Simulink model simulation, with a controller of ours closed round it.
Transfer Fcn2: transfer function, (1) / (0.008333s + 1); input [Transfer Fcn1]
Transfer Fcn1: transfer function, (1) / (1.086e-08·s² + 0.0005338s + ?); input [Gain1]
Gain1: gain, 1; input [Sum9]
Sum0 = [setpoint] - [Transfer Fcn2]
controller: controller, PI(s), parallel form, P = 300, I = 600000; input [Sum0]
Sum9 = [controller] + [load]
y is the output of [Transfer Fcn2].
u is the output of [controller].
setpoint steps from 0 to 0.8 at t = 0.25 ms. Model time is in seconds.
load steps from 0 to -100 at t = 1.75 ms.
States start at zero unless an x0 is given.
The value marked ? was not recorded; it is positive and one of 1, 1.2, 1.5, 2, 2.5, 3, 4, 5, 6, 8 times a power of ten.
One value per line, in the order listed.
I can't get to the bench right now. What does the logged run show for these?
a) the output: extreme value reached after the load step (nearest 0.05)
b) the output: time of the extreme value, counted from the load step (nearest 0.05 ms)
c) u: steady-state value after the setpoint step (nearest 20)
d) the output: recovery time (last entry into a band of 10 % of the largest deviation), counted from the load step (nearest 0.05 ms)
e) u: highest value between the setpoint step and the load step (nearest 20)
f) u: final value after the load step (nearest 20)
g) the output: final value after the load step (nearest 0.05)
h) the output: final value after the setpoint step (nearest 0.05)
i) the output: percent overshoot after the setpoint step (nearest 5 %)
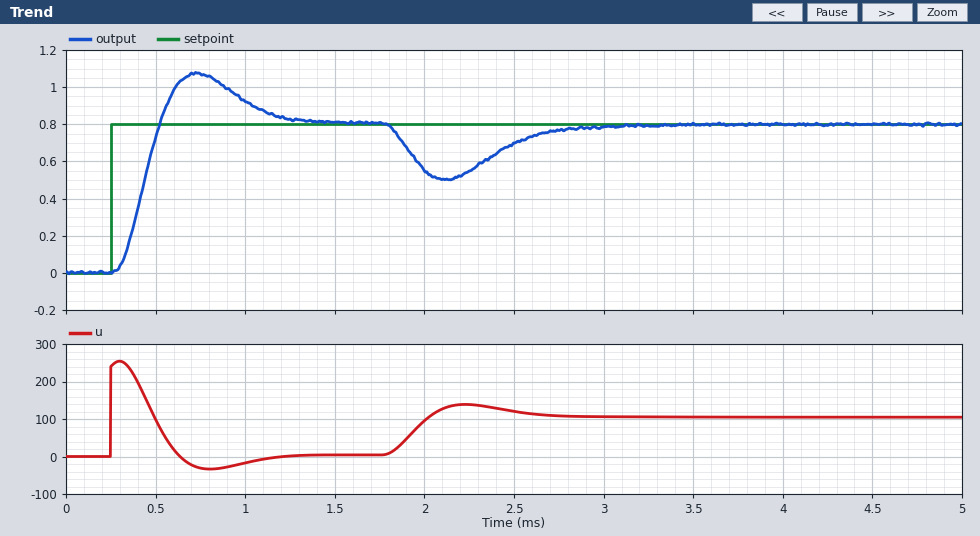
0.50
0.35 ms
0
1.00 ms
260
100
0.80
0.80
35 %
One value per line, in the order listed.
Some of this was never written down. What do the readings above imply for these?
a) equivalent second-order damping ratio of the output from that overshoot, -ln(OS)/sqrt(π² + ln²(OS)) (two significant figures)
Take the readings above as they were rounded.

0.32
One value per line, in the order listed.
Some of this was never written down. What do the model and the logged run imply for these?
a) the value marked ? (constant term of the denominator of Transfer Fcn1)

6
